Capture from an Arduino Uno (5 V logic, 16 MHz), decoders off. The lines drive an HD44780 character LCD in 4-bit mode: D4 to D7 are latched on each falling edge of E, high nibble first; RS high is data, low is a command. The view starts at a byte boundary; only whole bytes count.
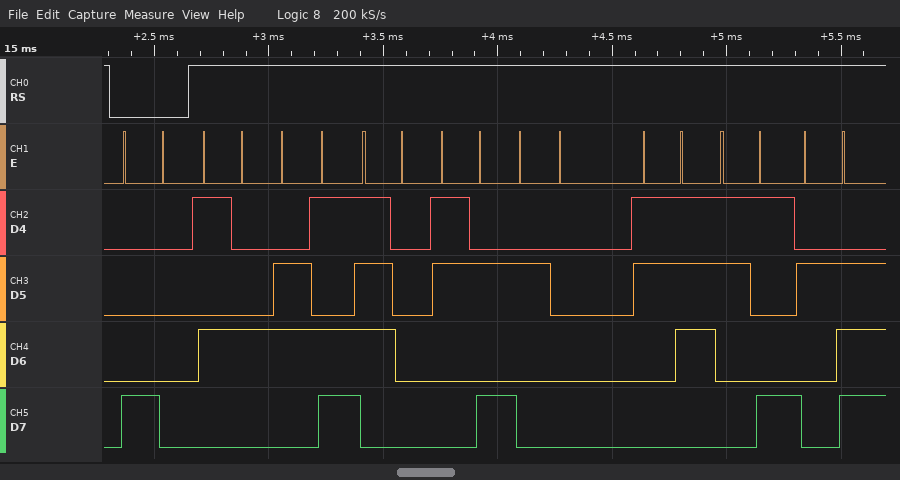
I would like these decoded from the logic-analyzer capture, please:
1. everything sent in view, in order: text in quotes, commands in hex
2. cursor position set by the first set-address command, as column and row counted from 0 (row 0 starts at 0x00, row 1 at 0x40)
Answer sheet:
0x80 "Tmp: 79."
column 0, row 0
